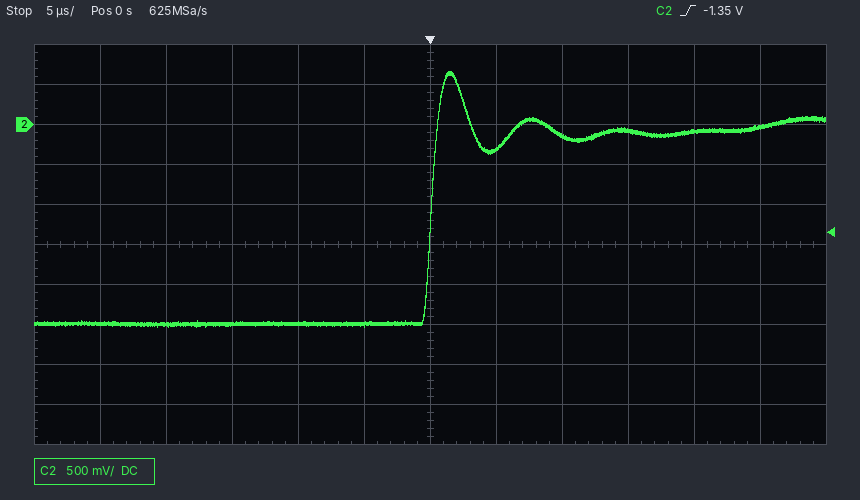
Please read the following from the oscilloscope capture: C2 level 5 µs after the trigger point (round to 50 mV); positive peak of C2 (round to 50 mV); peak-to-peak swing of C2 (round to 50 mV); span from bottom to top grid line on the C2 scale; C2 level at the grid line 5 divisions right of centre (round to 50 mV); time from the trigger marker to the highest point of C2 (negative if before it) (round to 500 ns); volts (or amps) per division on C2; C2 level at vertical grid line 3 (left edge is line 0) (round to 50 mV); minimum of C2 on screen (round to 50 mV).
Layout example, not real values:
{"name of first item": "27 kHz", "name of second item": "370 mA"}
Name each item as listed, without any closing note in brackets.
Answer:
{"C2 level 5 µs after the trigger point": "-300 mV", "positive peak of C2": "650 mV", "peak-to-peak swing of C2": "3.20 V", "span from bottom to top grid line on the C2 scale": "5 V", "C2 level at the grid line 5 divisions right of centre": "-50 mV", "time from the trigger marker to the highest point of C2 (negative if before it)": "+1.5 µs", "volts (or amps) per division on C2": "500 mV", "C2 level at vertical grid line 3 (left edge is line 0)": "-2.50 V", "minimum of C2 on screen": "-2.55 V"}
